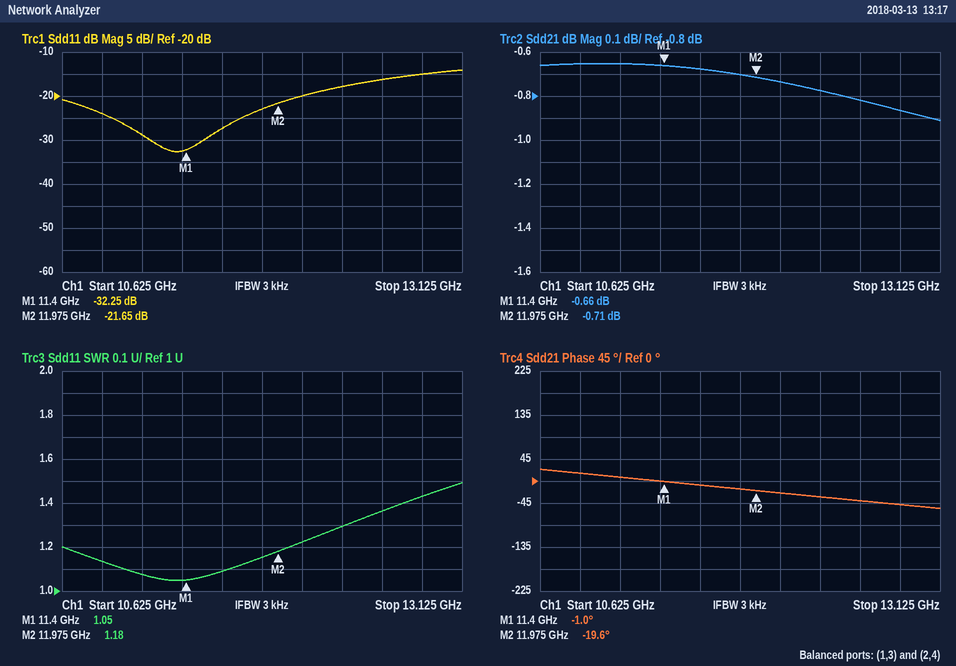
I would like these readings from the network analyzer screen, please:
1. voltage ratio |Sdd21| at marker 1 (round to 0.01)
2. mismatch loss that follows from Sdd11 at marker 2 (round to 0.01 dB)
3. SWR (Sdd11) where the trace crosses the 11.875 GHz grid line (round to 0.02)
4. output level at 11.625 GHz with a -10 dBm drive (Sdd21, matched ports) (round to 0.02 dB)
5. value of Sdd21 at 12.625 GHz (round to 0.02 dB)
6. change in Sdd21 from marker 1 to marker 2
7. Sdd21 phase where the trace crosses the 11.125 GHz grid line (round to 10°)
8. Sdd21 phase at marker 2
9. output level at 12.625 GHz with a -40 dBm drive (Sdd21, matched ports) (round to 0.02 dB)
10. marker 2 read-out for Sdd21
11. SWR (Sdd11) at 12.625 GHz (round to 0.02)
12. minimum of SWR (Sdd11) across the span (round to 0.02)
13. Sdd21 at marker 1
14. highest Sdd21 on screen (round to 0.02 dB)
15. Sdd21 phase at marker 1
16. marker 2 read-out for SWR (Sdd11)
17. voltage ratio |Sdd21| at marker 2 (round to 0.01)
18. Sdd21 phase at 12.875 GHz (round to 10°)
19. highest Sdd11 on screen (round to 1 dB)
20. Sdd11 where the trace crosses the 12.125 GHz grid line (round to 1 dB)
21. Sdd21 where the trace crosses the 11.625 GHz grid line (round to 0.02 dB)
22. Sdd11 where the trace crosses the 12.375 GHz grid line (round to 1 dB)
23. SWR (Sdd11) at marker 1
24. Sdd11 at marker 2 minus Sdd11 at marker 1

0.93
0.03 dB
1.16
-10.68 dBm
-0.82 dB
-0.05 dB
10°
-19.6°
-40.82 dBm
-0.71 dB
1.36
1.04
-0.66 dB
-0.66 dB
-1.0°
1.18
0.92
-50°
-14 dB
-20 dB
-0.68 dB
-18 dB
1.05
10.60 dB
